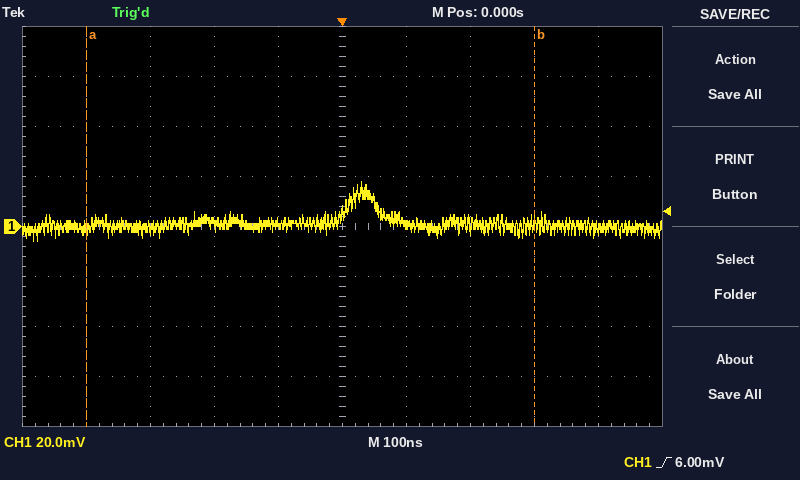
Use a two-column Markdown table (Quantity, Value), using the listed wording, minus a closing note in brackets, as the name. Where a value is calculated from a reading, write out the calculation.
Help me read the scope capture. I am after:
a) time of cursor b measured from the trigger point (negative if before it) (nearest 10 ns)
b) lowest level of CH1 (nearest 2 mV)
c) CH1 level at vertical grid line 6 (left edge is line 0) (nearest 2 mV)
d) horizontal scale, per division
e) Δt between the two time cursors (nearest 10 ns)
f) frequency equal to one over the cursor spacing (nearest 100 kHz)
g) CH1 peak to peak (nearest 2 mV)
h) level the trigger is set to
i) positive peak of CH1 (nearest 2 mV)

| Quantity | Value |
|---|---|
| time of cursor b measured from the trigger point (negative if before it) | +300 ns |
| lowest level of CH1 | -6 mV |
| CH1 level at vertical grid line 6 (left edge is line 0) | 0 mV |
| horizontal scale, per division | 100 ns |
| Δt between the two time cursors | 700 ns |
| frequency equal to one over the cursor spacing | 1 / 700 ns ≈ 1.4 MHz |
| CH1 peak to peak | 18 mV − (-6 mV) = 24 mV |
| level the trigger is set to | 6.00 mV |
| positive peak of CH1 | 18 mV |
